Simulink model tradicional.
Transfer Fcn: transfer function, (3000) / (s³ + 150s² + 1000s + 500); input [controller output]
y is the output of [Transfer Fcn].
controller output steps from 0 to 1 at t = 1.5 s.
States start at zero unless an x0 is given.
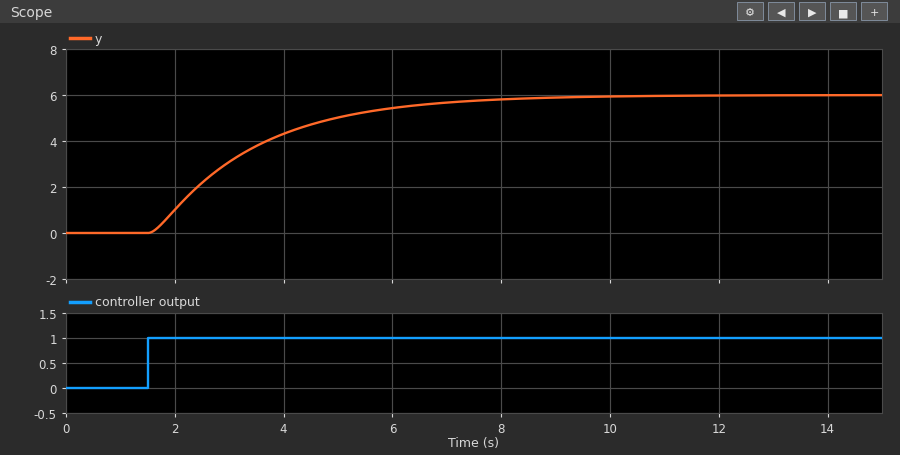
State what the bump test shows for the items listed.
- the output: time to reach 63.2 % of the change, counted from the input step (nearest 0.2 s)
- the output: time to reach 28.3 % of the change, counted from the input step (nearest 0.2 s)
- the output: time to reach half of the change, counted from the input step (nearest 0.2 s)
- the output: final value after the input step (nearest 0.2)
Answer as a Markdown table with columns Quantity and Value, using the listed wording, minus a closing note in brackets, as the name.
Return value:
| Quantity | Value |
|---|---|
| the output: time to reach 63.2 % of the change, counted from the input step | 2.0 s |
| the output: time to reach 28.3 % of the change, counted from the input step | 0.8 s |
| the output: time to reach half of the change, counted from the input step | 1.4 s |
| the output: final value after the input step | 6.0 |
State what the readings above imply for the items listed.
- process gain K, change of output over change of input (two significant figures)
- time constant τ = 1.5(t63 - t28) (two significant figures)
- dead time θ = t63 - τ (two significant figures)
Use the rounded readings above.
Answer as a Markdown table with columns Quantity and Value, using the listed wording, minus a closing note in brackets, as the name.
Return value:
| Quantity | Value |
|---|---|
| process gain K, change of output over change of input | 6.0 |
| time constant τ = 1.5(t63 - t28) | 1.8 s |
| dead time θ = t63 - τ | 0.20 s |
